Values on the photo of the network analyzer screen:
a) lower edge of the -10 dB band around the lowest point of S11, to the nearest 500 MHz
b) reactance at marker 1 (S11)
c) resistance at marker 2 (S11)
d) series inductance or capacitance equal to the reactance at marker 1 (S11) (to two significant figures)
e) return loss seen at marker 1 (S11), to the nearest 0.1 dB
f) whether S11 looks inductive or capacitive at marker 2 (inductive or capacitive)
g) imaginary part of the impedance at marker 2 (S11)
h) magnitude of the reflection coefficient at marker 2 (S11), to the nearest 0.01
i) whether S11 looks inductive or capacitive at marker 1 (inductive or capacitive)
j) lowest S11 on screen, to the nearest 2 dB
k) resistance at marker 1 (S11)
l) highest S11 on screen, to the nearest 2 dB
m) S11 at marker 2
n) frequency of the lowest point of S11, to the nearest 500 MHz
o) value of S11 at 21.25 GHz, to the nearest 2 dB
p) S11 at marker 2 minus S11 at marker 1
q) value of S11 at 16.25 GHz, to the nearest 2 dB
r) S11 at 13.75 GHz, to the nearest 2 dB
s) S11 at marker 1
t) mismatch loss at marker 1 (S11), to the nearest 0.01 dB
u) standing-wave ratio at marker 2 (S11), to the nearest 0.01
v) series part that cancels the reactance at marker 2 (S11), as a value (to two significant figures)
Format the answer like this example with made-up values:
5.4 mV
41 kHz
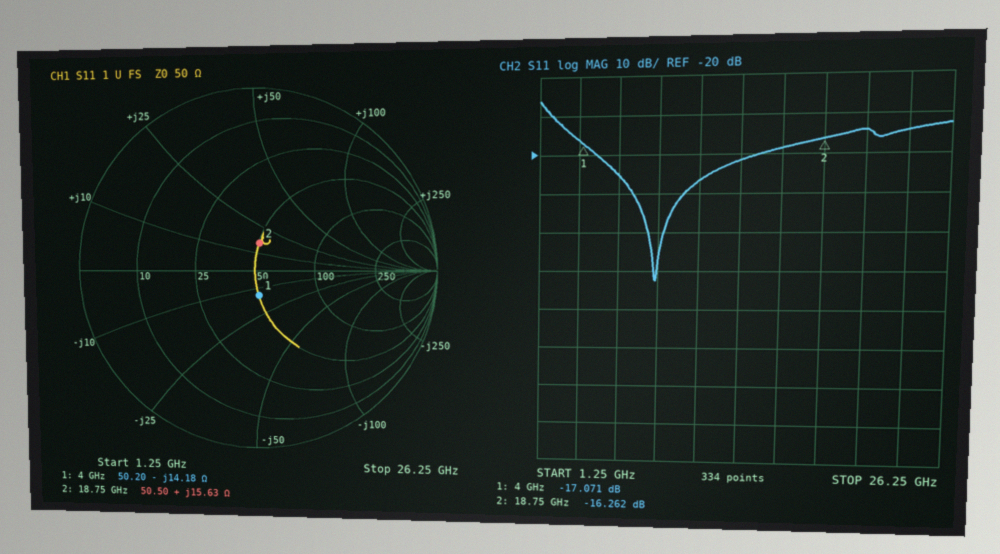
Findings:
2.0 GHz
-14.18 Ω
50.50 Ω
2.8 pF
17.1 dB
inductive
+15.63 Ω
0.15
capacitive
-52 dB
50.20 Ω
-6 dB
-16.262 dB
8.5 GHz
-14 dB
0.809 dB
-18 dB
-22 dB
-17.071 dB
0.09 dB
1.36
540 fF
